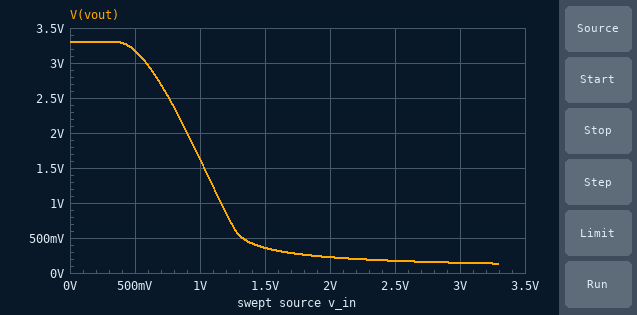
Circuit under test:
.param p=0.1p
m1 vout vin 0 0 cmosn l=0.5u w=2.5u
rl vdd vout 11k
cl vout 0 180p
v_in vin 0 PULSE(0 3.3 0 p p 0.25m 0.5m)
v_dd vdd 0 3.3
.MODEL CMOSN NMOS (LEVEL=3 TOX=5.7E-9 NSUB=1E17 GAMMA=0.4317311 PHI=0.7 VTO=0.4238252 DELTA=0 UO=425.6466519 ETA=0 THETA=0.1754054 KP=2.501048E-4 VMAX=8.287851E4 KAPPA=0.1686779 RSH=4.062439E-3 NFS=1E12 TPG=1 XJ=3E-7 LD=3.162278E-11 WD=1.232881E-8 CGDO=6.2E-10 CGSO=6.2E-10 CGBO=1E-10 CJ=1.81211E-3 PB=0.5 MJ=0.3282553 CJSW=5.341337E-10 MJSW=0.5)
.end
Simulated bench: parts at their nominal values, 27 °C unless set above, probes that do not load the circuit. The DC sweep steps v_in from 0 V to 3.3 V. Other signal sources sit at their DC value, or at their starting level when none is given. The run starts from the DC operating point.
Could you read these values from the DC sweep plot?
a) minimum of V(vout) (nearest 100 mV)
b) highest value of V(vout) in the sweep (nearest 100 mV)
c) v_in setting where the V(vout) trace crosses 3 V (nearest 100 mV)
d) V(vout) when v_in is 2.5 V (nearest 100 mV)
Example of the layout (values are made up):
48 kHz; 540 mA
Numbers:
100 mV; 3.3 V; 600 mV; 200 mV
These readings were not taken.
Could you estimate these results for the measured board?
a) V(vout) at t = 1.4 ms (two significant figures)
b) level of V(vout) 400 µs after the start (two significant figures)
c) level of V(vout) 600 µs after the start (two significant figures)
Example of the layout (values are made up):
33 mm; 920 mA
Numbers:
3.3 V; 3.3 V; 130 mV
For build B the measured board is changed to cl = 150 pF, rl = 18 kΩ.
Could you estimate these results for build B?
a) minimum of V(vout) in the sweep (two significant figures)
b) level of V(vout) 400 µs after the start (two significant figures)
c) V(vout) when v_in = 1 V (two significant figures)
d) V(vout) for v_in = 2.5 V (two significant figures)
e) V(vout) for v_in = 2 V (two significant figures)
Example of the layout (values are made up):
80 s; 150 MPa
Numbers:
80 mV; 3.3 V; 710 mV; 100 mV; 130 mV
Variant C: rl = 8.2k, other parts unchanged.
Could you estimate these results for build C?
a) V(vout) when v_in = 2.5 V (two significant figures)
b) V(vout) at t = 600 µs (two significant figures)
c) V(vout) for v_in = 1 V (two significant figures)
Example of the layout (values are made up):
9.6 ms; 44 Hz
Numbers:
240 mV; 180 mV; 2.0 V
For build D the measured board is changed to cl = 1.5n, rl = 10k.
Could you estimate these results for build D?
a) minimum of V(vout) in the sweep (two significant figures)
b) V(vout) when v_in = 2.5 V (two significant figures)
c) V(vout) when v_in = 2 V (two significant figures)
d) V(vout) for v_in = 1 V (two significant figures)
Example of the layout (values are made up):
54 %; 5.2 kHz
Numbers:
150 mV; 190 mV; 250 mV; 1.8 V
